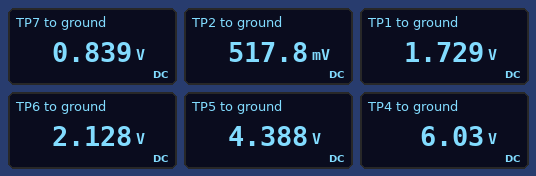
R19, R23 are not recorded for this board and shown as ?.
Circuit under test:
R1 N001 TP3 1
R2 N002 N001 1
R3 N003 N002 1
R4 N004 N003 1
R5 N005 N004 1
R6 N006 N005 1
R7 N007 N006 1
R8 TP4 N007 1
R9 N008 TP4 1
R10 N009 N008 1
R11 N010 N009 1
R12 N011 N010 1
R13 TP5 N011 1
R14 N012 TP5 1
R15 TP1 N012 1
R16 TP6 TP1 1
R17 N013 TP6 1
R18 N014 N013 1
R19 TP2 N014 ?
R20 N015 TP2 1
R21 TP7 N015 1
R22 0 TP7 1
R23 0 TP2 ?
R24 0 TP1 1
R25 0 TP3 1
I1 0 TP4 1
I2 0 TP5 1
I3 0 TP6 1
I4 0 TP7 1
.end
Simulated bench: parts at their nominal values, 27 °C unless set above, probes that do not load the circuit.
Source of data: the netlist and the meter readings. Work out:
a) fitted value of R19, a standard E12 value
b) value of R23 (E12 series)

0.68 Ω
0.68 Ω
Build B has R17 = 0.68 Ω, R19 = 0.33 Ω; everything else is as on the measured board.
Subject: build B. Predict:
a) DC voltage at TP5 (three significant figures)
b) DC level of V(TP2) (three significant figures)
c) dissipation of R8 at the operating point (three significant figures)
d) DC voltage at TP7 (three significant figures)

4.31 V
567 mV
443 mW
856 mV
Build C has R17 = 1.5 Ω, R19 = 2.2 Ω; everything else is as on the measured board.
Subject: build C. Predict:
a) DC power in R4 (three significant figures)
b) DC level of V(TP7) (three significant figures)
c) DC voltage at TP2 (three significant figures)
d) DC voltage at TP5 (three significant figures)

463 mW
808 mV
424 mV
4.53 V
